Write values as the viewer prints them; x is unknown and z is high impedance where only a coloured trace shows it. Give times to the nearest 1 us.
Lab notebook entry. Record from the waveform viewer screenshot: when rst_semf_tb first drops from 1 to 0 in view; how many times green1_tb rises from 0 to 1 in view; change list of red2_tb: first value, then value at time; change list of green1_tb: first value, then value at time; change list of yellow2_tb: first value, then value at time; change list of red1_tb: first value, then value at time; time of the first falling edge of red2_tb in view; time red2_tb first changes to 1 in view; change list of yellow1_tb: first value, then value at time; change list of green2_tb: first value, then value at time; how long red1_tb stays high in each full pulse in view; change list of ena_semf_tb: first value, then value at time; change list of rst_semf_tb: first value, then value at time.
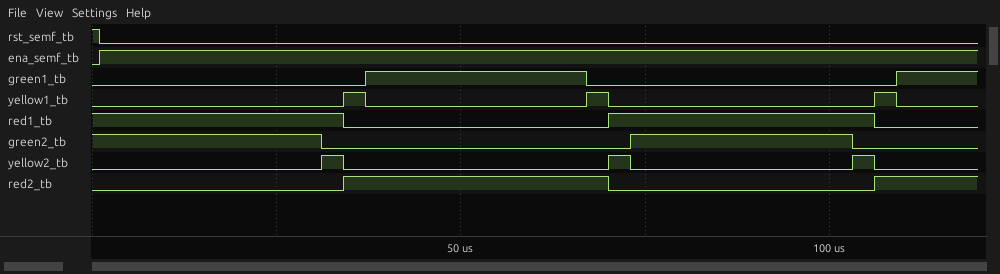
1 us
2
0, 1 at 34 us, 0 at 70 us, 1 at 106 us
0, 1 at 37 us, 0 at 67 us, 1 at 109 us
0, 1 at 31 us, 0 at 34 us, 1 at 70 us, 0 at 73 us, 1 at 103 us, 0 at 106 us
1, 0 at 34 us, 1 at 70 us, 0 at 106 us
70 us
34 us
0, 1 at 34 us, 0 at 37 us, 1 at 67 us, 0 at 70 us, 1 at 106 us, 0 at 109 us
1, 0 at 31 us, 1 at 73 us, 0 at 103 us
36 us
0, 1 at 1 us
1, 0 at 1 us
